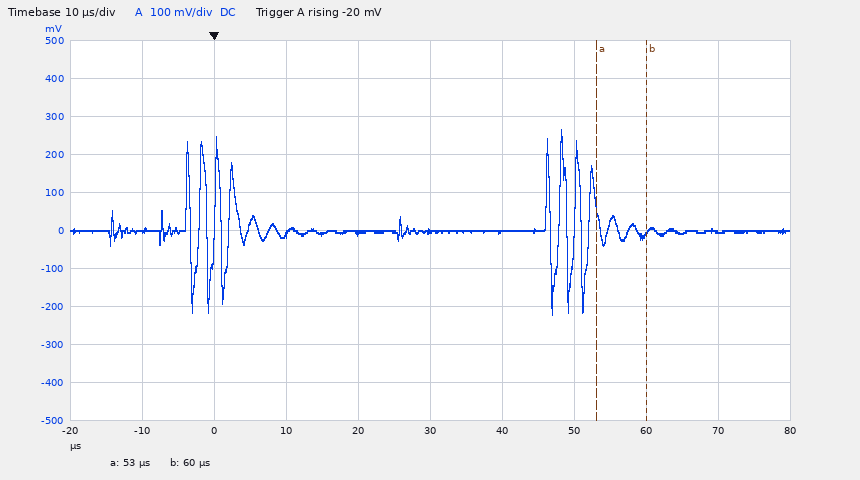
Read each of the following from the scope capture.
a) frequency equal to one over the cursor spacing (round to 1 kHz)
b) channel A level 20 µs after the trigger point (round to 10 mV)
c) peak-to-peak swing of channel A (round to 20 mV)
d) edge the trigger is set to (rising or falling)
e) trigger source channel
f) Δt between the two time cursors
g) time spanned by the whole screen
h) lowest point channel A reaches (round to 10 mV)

143 kHz
-10 mV
480 mV
rising
channel A
7 µs
100 µs
-220 mV
